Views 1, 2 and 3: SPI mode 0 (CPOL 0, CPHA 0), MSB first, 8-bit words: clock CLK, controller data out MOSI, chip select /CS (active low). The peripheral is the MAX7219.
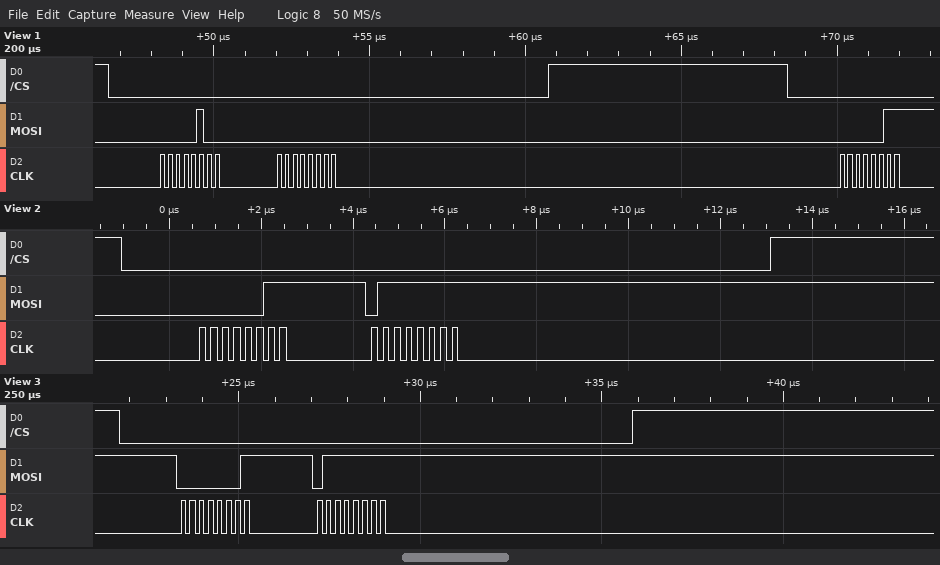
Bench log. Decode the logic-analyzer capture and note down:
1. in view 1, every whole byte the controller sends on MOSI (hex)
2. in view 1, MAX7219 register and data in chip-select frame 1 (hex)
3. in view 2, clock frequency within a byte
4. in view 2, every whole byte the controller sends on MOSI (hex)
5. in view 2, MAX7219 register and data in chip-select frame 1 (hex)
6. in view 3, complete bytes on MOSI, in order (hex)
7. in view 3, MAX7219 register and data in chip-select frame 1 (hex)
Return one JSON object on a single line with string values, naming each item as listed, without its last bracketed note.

{"in view 1, every whole byte the controller sends on MOSI": "04 00 03", "in view 1, MAX7219 register and data in chip-select frame 1": "register 0x4, data 0x00", "in view 2, clock frequency within a byte": "4 MHz", "in view 2, every whole byte the controller sends on MOSI": "03 7F", "in view 2, MAX7219 register and data in chip-select frame 1": "register 0x3, data 0x7F", "in view 3, complete bytes on MOSI, in order": "01 7F", "in view 3, MAX7219 register and data in chip-select frame 1": "register 0x1, data 0x7F"}
